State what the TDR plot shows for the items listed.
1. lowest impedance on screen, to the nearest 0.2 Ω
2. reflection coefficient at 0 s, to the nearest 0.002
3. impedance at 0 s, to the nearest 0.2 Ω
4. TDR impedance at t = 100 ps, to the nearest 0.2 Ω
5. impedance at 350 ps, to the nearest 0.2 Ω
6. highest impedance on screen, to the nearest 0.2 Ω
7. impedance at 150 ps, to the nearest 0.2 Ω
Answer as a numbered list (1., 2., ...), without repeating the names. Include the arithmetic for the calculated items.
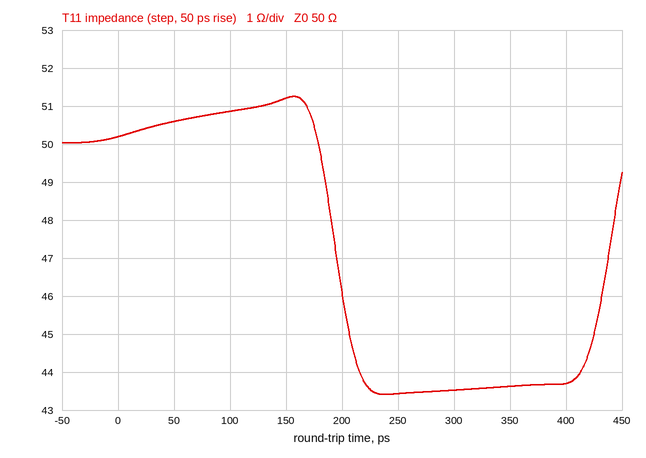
1. 43.4 Ω
2. (50.2 − 50)/(50.2 + 50) ≈ +0.002
3. 50.2 Ω
4. 50.8 Ω
5. 43.6 Ω
6. 51.2 Ω
7. 51.2 Ω
